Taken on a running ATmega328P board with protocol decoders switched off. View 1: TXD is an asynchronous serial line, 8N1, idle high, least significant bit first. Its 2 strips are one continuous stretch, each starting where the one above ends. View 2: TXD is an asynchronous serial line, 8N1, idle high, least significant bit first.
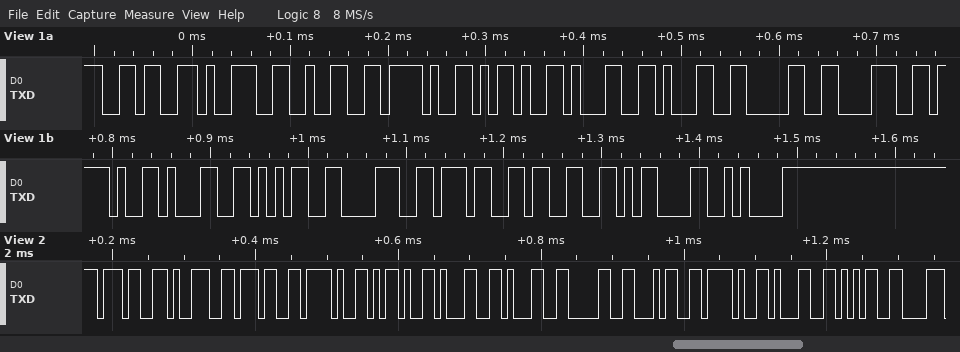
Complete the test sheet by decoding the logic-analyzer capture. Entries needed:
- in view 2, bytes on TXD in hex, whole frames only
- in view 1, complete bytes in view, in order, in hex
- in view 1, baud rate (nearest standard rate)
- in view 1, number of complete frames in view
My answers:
0x37 0x39 0x37 0x2F 0x2D 0x31 0x31 0x30 0x34 0x2F 0x31 0x35
36 39 32 2F 2D 31 31 30 38 2F 31 35 38 37 33 0D 0A
115200 baud
17
